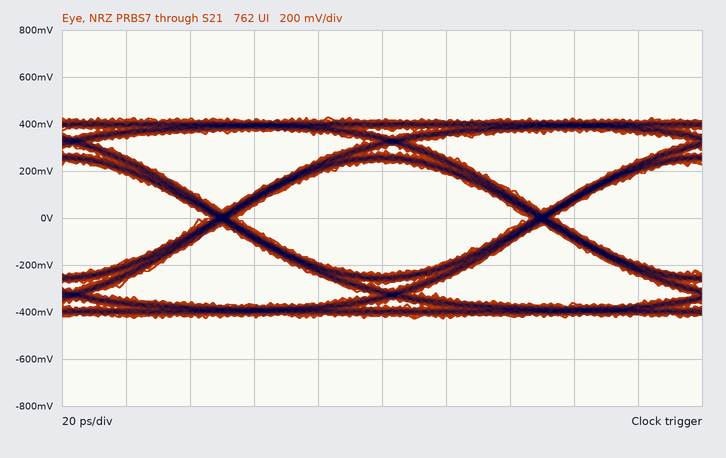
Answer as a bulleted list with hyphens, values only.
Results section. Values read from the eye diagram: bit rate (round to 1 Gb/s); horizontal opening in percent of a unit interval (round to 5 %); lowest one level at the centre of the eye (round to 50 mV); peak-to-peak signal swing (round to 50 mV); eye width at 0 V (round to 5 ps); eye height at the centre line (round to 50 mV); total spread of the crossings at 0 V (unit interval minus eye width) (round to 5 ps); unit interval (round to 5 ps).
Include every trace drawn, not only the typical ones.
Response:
- 10 Gb/s
- 90 %
- 250 mV
- 850 mV
- 90 ps
- 500 mV
- 10 ps
- 100 ps
